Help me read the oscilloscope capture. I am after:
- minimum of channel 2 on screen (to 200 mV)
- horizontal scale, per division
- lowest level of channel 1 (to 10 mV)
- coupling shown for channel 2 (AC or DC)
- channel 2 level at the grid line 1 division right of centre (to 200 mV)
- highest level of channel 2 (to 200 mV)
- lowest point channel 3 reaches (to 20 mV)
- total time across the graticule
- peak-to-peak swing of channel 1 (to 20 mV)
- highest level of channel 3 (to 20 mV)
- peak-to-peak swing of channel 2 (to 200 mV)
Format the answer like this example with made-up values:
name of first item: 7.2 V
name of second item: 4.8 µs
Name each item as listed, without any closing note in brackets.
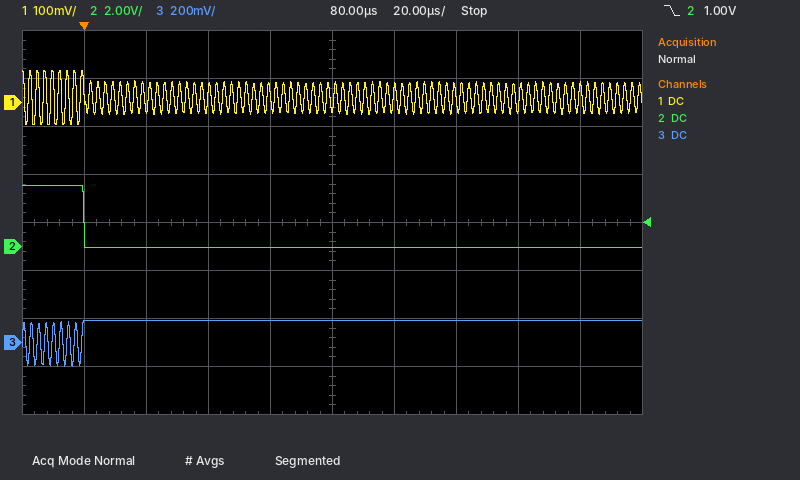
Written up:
minimum of channel 2 on screen: 0.0 V
horizontal scale, per division: 20 µs
lowest level of channel 1: -50 mV
coupling shown for channel 2: DC
channel 2 level at the grid line 1 division right of centre: 0.0 V
highest level of channel 2: 2.6 V
lowest point channel 3 reaches: -100 mV
total time across the graticule: 200 µs
peak-to-peak swing of channel 1: 120 mV
highest level of channel 3: 100 mV
peak-to-peak swing of channel 2: 2.6 V
